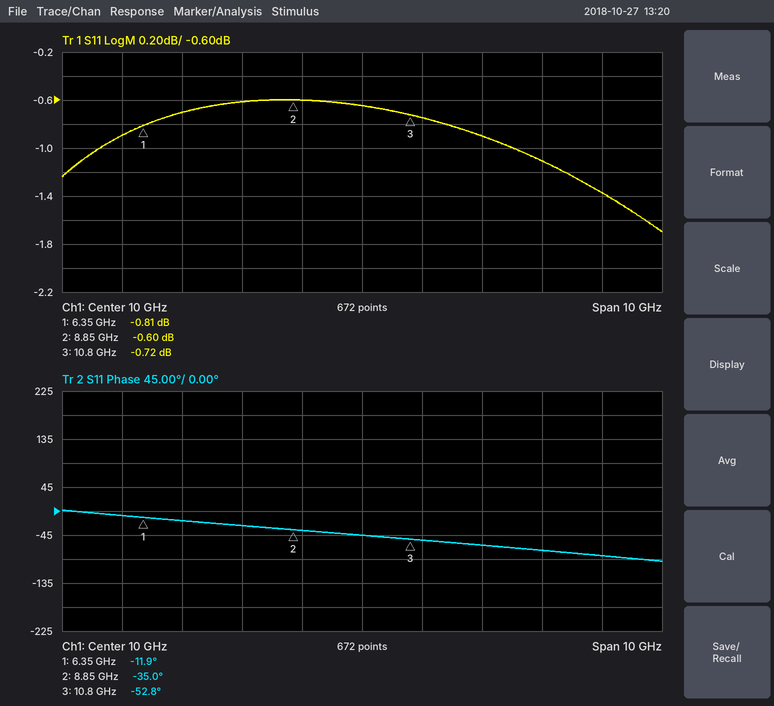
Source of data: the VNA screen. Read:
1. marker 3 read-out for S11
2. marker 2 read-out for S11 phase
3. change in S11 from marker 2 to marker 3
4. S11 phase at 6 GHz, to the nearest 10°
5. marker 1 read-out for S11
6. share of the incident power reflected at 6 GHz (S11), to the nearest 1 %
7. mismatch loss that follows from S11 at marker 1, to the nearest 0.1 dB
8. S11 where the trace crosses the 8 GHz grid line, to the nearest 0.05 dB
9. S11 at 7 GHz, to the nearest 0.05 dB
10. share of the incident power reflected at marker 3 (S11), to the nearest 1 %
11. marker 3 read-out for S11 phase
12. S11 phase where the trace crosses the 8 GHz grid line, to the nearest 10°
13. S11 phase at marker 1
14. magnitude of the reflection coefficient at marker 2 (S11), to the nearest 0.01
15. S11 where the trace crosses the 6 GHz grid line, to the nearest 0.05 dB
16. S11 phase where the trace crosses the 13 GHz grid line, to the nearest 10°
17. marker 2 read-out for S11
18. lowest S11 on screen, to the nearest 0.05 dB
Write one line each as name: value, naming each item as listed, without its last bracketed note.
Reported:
marker 3 read-out for S11: -0.72 dB
marker 2 read-out for S11 phase: -35.0°
change in S11 from marker 2 to marker 3: -0.12 dB
S11 phase at 6 GHz, to the nearest 10°: -10°
marker 1 read-out for S11: -0.81 dB
share of the incident power reflected at 6 GHz (S11), to the nearest 1 %: 81 %
mismatch loss that follows from S11 at marker 1, to the nearest 0.1 dB: 7.7 dB
S11 where the trace crosses the 8 GHz grid line, to the nearest 0.05 dB: -0.60 dB
S11 at 7 GHz, to the nearest 0.05 dB: -0.70 dB
share of the incident power reflected at marker 3 (S11), to the nearest 1 %: 85 %
marker 3 read-out for S11 phase: -52.8°
S11 phase where the trace crosses the 8 GHz grid line, to the nearest 10°: -30°
S11 phase at marker 1: -11.9°
magnitude of the reflection coefficient at marker 2 (S11), to the nearest 0.01: 0.93
S11 where the trace crosses the 6 GHz grid line, to the nearest 0.05 dB: -0.90 dB
S11 phase where the trace crosses the 13 GHz grid line, to the nearest 10°: -70°
marker 2 read-out for S11: -0.60 dB
lowest S11 on screen, to the nearest 0.05 dB: -1.70 dB
